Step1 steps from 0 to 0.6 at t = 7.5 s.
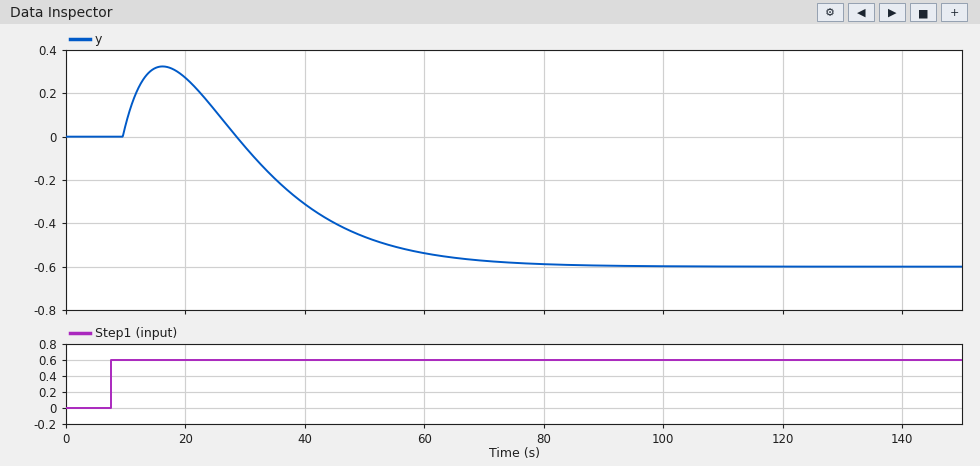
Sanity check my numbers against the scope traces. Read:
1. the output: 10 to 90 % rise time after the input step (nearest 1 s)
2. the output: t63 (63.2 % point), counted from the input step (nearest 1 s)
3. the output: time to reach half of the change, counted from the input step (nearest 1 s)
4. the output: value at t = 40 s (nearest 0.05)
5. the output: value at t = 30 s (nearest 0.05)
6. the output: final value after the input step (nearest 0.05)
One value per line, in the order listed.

30 s
36 s
32 s
-0.30
-0.05
-0.60
